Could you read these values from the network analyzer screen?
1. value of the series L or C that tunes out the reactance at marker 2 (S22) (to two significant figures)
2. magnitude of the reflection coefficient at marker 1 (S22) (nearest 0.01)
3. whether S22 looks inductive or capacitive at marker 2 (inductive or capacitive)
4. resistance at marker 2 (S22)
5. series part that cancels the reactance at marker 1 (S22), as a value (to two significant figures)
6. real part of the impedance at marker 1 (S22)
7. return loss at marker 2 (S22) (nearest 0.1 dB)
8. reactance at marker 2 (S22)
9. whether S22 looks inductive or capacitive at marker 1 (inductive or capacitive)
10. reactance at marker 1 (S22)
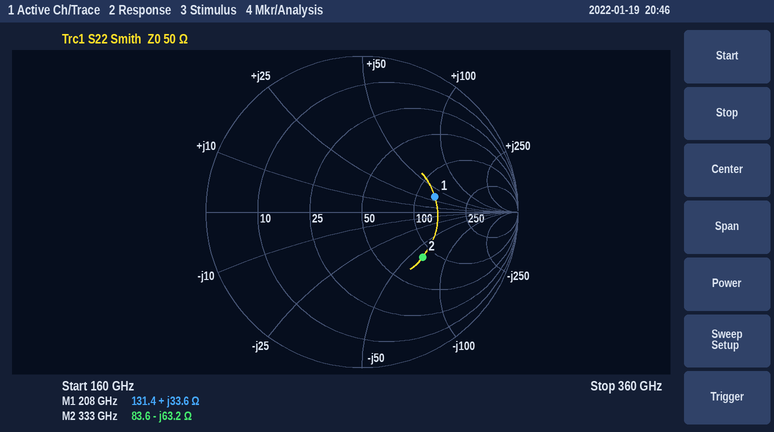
30 pH
0.48
capacitive
83.6 Ω
23 fF
131.4 Ω
6.3 dB
-63.2 Ω
inductive
+33.6 Ω
